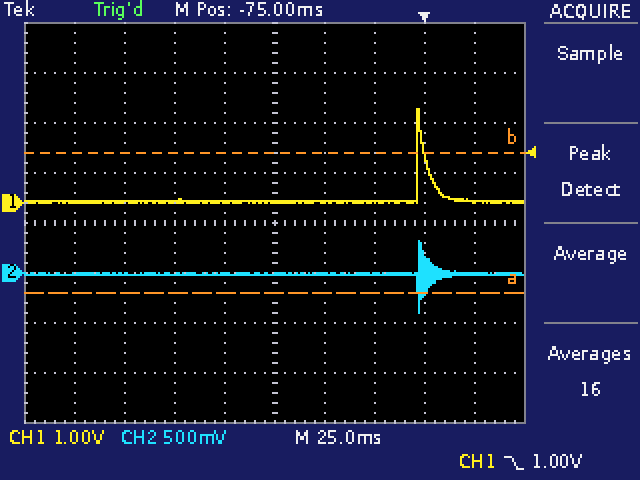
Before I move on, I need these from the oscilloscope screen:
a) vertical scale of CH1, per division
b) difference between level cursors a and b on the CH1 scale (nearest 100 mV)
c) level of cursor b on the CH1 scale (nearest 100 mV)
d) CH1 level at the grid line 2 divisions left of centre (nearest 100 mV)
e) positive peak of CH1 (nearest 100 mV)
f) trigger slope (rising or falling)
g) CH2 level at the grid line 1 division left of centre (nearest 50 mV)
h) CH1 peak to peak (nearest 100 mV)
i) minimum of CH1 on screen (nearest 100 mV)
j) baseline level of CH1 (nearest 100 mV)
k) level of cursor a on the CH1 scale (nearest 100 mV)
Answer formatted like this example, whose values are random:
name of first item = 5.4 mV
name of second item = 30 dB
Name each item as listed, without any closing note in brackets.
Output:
vertical scale of CH1, per division = 1 V
difference between level cursors a and b on the CH1 scale = 2.8 V
level of cursor b on the CH1 scale = 1.0 V
CH1 level at the grid line 2 divisions left of centre = 0.0 V
positive peak of CH1 = 1.9 V
trigger slope = falling
CH2 level at the grid line 1 division left of centre = 0 mV
CH1 peak to peak = 1.9 V
minimum of CH1 on screen = 0.0 V
baseline level of CH1 = 0.0 V
level of cursor a on the CH1 scale = -1.8 V
